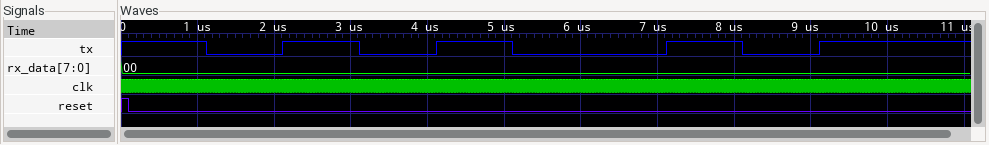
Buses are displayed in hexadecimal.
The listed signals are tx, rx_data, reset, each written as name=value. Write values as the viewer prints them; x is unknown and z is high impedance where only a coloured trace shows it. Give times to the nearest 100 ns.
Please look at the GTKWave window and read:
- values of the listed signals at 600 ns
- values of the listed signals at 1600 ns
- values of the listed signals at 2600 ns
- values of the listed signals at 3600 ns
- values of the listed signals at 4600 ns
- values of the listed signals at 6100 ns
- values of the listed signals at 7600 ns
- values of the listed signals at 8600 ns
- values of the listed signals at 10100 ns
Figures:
tx=1, rx_data=00, reset=0
tx=0, rx_data=00, reset=0
tx=1, rx_data=00, reset=0
tx=0, rx_data=00, reset=0
tx=1, rx_data=00, reset=0
tx=0, rx_data=00, reset=0
tx=1, rx_data=00, reset=0
tx=0, rx_data=00, reset=0
tx=1, rx_data=00, reset=0
